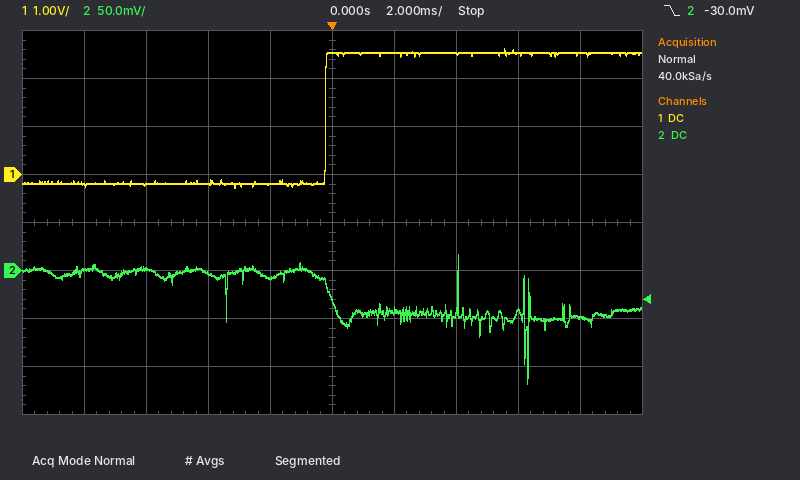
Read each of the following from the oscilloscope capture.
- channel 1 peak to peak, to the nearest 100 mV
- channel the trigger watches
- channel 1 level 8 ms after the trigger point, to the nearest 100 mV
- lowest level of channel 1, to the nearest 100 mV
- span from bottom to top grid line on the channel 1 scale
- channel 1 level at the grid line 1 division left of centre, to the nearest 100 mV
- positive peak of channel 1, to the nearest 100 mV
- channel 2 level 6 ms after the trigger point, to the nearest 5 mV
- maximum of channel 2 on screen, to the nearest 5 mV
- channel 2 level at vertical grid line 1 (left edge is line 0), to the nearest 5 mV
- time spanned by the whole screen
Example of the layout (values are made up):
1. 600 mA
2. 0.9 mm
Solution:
1. 2.9 V
2. channel 2
3. 2.5 V
4. -300 mV
5. 8 V
6. -200 mV
7. 2.6 V
8. -45 mV
9. 15 mV
10. 0 mV
11. 20 ms
